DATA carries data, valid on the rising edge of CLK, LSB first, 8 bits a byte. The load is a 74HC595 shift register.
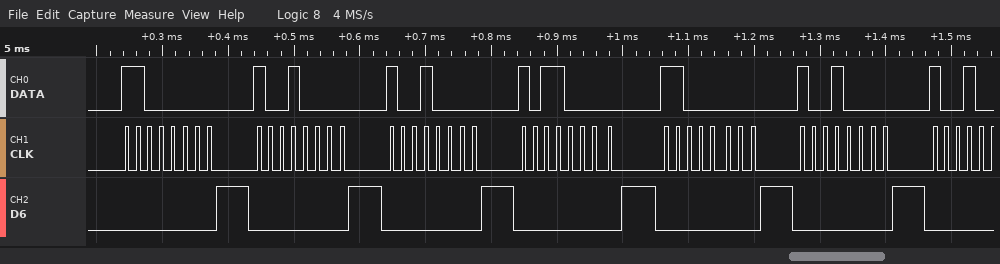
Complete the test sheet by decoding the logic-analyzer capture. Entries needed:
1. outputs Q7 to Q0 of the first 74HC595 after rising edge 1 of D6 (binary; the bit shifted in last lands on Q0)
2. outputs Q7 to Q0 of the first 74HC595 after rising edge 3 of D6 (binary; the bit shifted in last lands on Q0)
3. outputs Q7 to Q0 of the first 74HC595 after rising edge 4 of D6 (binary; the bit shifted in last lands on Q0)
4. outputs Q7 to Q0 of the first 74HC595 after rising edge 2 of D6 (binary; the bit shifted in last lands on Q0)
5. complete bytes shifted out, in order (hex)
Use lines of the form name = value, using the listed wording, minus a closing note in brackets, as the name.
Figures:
outputs Q7 to Q0 of the first 74HC595 after rising edge 1 of D6 = 11000000
outputs Q7 to Q0 of the first 74HC595 after rising edge 3 of D6 = 10010000
outputs Q7 to Q0 of the first 74HC595 after rising edge 4 of D6 = 10110000
outputs Q7 to Q0 of the first 74HC595 after rising edge 2 of D6 = 10010000
complete bytes shifted out, in order = 0x03 0x09 0x09 0x0D 0x03 0x09
